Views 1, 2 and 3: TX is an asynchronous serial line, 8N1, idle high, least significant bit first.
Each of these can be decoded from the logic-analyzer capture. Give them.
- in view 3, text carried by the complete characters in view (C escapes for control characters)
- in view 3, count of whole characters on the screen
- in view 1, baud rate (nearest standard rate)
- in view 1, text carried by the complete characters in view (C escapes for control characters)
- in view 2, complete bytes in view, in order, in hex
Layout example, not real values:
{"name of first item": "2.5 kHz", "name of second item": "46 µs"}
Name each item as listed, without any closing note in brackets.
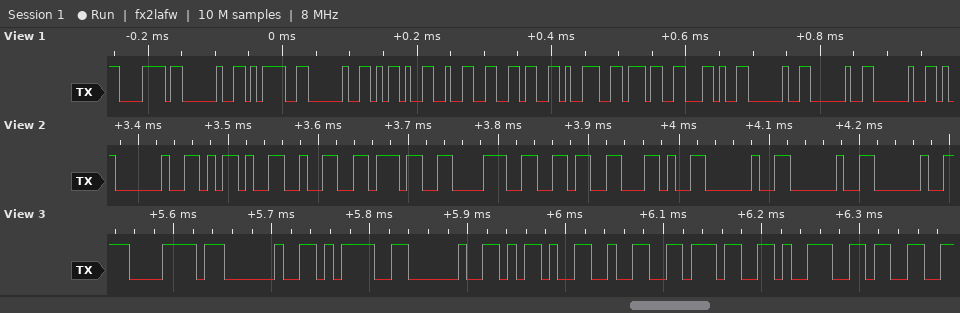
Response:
{"in view 3, text carried by the complete characters in view": "\"x = -2793\"", "in view 3, count of whole characters on the screen": "9", "in view 1, baud rate": "115200 baud", "in view 1, text carried by the complete characters in view": "\"x = -2697,   \"", "in view 2, complete bytes in view, in order, in hex": "0x20 0x2D 0x32 0x37 0x38 0x36 0x2C 0x20 0x20 0x20"}
